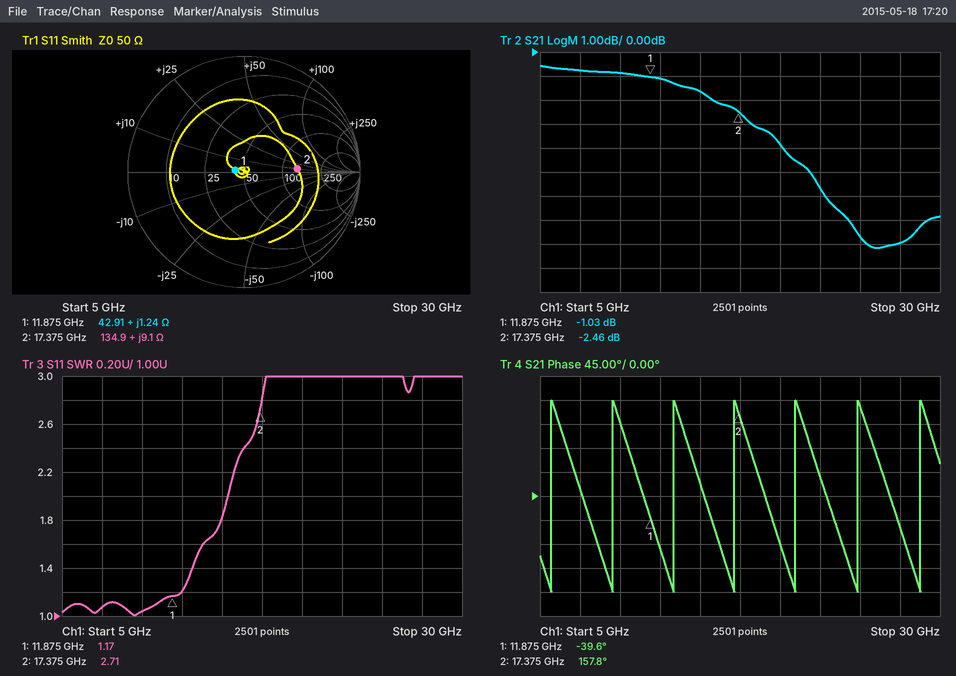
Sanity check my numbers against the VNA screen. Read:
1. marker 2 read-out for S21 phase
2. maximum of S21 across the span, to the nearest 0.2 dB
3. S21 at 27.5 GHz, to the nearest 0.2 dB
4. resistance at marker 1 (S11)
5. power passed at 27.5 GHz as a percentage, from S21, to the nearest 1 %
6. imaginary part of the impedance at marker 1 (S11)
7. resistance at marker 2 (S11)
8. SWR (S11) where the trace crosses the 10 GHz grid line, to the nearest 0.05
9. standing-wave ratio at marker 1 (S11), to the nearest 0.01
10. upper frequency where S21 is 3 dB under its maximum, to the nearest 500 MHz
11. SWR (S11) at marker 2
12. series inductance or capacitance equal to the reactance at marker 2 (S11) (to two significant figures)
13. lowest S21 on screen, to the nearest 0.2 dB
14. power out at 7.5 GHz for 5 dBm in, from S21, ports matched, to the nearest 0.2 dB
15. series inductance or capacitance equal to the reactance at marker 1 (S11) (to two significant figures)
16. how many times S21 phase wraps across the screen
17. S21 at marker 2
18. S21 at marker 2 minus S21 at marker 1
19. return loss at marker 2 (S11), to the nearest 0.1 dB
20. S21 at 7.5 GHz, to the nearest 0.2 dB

157.8°
-0.6 dB
-8.0 dB
42.91 Ω
16 %
+1.24 Ω
134.9 Ω
1.05
1.17
19.5 GHz
2.71
83 pH
-8.2 dB
4.2 dBm
17 pH
7
-2.46 dB
-1.43 dB
6.7 dB
-0.8 dB
